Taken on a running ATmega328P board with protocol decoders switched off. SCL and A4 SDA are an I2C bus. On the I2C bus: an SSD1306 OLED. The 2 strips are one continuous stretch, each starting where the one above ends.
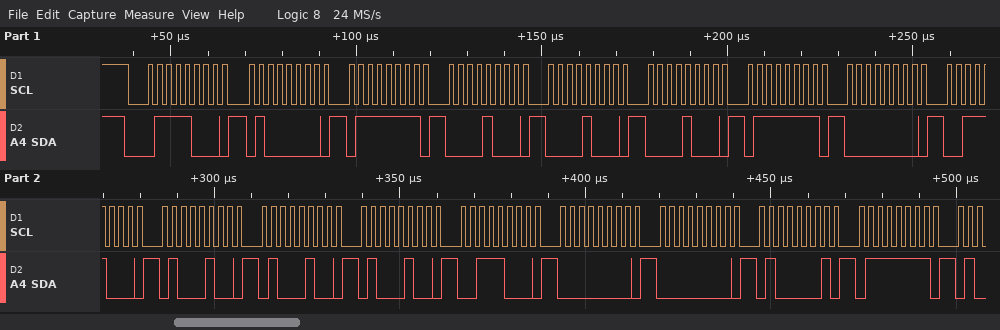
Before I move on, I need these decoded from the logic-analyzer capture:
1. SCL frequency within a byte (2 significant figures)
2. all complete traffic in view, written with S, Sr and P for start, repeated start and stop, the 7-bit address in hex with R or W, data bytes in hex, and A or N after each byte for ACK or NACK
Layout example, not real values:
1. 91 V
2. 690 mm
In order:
1. 400 kHz
2. S 3CW A 40 A 7F A 08 A 08 A 08 A 7F A 00 A 38 A 44 A 44 A 44 A 38 A 00 A 00 A 41 A 7F A
